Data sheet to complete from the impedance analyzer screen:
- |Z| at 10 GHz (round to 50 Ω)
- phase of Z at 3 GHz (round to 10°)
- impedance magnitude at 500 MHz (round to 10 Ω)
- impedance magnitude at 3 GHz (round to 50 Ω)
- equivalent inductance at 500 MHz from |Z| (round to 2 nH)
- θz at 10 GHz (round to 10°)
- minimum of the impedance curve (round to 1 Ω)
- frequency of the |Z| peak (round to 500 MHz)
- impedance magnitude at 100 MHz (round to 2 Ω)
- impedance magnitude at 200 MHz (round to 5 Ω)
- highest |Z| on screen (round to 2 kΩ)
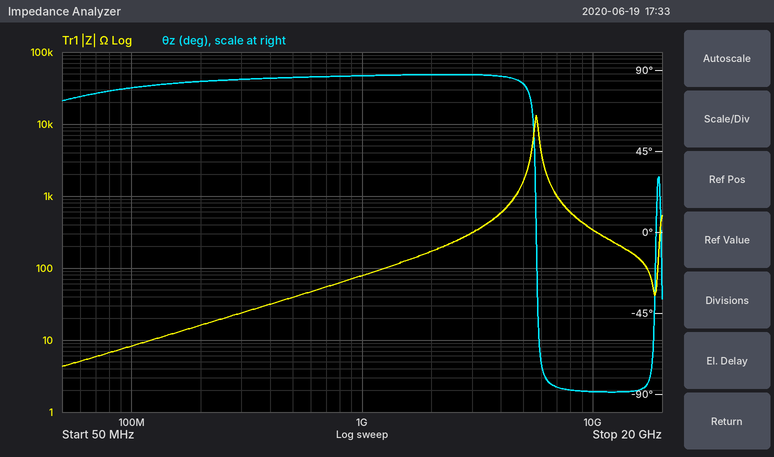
350 Ω
90°
40 Ω
300 Ω
12 nH
-90°
4 Ω
5.5 GHz
8 Ω
15 Ω
14 kΩ
